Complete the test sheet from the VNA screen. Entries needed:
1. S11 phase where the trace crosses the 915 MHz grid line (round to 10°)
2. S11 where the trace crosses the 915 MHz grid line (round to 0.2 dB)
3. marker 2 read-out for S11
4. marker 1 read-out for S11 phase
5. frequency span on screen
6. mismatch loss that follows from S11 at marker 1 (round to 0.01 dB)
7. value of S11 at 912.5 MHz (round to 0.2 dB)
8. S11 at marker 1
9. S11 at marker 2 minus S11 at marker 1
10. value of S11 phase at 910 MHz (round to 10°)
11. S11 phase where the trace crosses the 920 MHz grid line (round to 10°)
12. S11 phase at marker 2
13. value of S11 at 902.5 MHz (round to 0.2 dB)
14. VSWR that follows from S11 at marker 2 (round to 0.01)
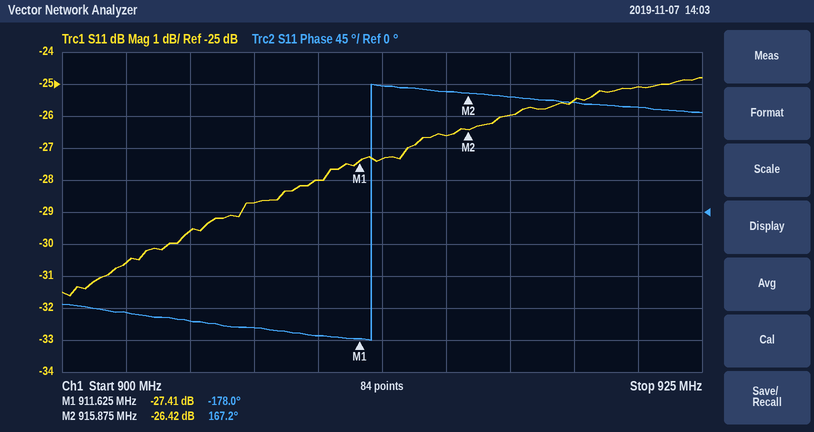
170°
-26.6 dB
-26.42 dB
-178.0°
25 MHz
0.01 dB
-27.4 dB
-27.41 dB
0.99 dB
-170°
150°
167.2°
-30.6 dB
1.10
